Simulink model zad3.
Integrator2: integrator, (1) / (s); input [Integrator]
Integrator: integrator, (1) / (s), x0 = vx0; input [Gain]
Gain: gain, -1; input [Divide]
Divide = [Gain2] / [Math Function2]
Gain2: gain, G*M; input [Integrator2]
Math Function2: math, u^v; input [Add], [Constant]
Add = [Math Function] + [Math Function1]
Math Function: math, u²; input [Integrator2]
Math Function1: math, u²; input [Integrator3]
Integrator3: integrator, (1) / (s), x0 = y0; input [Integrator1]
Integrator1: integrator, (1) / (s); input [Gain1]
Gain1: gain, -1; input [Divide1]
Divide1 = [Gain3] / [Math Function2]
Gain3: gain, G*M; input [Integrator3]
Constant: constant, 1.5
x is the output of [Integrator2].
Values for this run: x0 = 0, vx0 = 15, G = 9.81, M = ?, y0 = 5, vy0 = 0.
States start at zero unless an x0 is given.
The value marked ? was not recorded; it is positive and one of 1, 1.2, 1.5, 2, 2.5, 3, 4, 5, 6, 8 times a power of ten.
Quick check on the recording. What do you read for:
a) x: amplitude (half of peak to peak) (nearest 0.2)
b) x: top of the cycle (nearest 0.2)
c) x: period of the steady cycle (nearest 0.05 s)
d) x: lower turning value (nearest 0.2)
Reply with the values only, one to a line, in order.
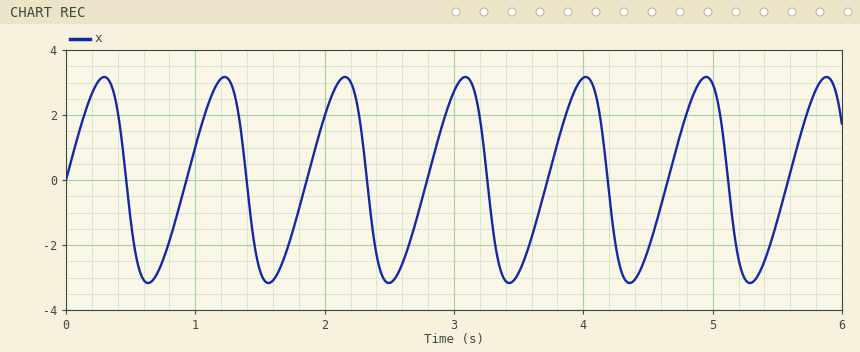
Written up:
3.2
3.2
0.95 s
-3.2
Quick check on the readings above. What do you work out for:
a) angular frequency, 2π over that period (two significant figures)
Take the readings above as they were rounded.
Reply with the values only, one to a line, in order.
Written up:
6.6 rad/s
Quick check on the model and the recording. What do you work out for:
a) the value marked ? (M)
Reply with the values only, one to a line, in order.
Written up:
200
